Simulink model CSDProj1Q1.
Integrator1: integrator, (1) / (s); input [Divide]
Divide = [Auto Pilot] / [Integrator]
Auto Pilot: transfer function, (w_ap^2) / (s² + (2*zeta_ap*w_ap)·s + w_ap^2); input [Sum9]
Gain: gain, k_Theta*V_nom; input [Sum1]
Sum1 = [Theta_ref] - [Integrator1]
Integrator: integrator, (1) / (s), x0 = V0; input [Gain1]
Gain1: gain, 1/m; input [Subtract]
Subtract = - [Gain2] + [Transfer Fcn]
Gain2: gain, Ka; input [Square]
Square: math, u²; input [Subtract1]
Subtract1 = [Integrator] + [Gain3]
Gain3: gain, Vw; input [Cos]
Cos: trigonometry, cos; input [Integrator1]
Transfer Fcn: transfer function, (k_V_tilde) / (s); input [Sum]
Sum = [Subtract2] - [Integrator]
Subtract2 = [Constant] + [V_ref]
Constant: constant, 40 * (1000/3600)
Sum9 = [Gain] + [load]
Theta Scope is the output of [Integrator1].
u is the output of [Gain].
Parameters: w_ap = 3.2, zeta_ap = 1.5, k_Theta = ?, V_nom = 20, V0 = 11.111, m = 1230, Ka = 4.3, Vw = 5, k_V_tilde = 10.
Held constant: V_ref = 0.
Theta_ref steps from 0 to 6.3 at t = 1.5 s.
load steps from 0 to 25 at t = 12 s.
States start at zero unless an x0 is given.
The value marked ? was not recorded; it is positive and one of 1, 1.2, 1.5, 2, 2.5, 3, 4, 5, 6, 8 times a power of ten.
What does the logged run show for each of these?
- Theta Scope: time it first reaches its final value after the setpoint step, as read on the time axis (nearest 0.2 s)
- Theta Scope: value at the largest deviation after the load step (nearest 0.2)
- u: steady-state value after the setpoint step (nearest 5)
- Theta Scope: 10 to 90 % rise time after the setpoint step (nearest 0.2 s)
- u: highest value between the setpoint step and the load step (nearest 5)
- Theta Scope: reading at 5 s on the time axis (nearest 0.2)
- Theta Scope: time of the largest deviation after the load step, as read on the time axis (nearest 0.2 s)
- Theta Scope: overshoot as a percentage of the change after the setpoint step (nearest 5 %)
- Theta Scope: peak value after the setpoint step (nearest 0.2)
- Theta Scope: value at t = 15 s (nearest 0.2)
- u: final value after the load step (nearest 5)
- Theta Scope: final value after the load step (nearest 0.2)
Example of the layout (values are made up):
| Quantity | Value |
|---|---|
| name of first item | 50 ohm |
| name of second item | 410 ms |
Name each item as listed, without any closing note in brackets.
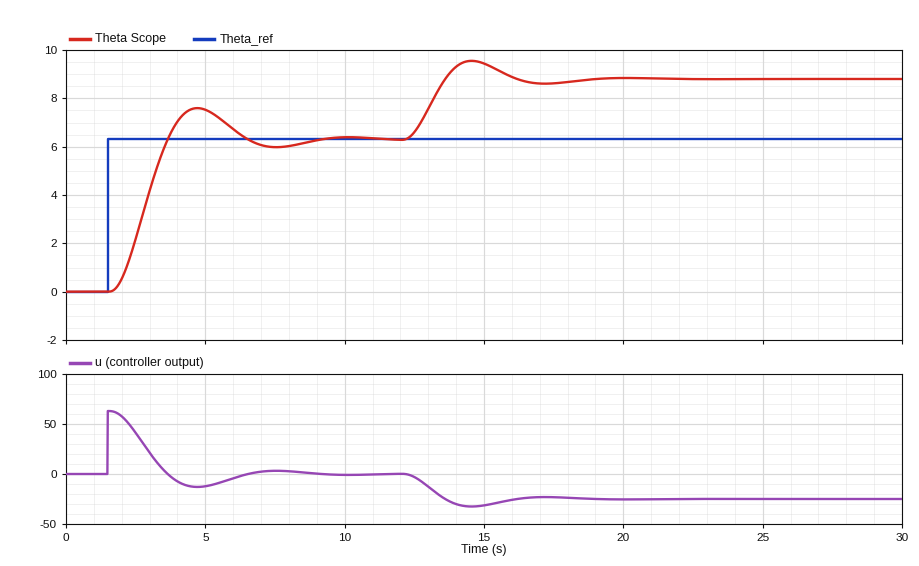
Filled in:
| Quantity | Value |
|---|---|
| Theta Scope: time it first reaches its final value after the setpoint step, as read on the time axis | 3.6 s |
| Theta Scope: value at the largest deviation after the load step | 9.6 |
| u: steady-state value after the setpoint step | 0 |
| Theta Scope: 10 to 90 % rise time after the setpoint step | 1.4 s |
| u: highest value between the setpoint step and the load step | 65 |
| Theta Scope: reading at 5 s on the time axis | 7.6 |
| Theta Scope: time of the largest deviation after the load step, as read on the time axis | 14.6 s |
| Theta Scope: overshoot as a percentage of the change after the setpoint step | 20 % |
| Theta Scope: peak value after the setpoint step | 7.6 |
| Theta Scope: value at t = 15 s | 9.4 |
| u: final value after the load step | -25 |
| Theta Scope: final value after the load step | 8.8 |
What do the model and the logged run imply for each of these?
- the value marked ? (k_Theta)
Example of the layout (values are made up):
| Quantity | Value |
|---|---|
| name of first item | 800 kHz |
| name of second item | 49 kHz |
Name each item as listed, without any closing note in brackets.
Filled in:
| Quantity | Value |
|---|---|
| the value marked ? | 0.5 |
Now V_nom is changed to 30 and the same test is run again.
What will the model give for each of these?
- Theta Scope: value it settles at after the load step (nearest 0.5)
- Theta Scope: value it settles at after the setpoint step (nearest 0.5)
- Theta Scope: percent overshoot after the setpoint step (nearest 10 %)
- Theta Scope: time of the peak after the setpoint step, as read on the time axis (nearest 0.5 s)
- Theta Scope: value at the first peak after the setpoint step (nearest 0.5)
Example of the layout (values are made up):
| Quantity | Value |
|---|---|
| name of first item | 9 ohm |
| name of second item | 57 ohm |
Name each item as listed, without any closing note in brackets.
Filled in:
| Quantity | Value |
|---|---|
| Theta Scope: value it settles at after the load step | 8.0 |
| Theta Scope: value it settles at after the setpoint step | 6.5 |
| Theta Scope: percent overshoot after the setpoint step | 30 % |
| Theta Scope: time of the peak after the setpoint step, as read on the time axis | 4.0 s |
| Theta Scope: value at the first peak after the setpoint step | 8.5 |
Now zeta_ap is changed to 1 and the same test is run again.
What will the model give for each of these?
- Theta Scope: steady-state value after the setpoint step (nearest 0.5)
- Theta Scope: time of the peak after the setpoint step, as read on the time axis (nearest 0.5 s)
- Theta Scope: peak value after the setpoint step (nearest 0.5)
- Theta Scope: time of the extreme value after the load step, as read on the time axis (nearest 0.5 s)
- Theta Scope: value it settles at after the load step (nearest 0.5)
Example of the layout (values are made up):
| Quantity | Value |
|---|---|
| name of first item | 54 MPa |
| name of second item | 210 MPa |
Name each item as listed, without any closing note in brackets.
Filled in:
| Quantity | Value |
|---|---|
| Theta Scope: steady-state value after the setpoint step | 6.5 |
| Theta Scope: time of the peak after the setpoint step, as read on the time axis | 4.0 s |
| Theta Scope: peak value after the setpoint step | 7.0 |
| Theta Scope: time of the extreme value after the load step, as read on the time axis | 14.0 s |
| Theta Scope: value it settles at after the load step | 9.0 |
